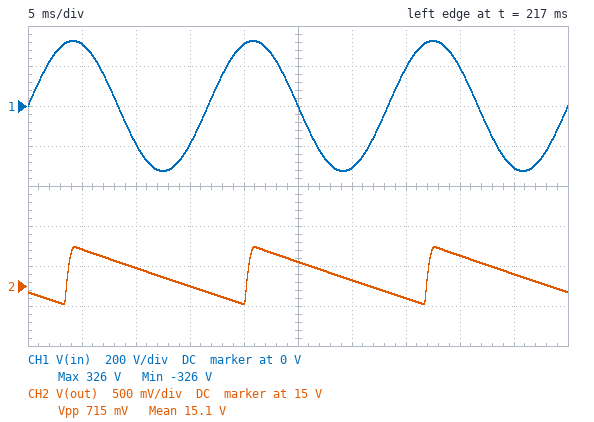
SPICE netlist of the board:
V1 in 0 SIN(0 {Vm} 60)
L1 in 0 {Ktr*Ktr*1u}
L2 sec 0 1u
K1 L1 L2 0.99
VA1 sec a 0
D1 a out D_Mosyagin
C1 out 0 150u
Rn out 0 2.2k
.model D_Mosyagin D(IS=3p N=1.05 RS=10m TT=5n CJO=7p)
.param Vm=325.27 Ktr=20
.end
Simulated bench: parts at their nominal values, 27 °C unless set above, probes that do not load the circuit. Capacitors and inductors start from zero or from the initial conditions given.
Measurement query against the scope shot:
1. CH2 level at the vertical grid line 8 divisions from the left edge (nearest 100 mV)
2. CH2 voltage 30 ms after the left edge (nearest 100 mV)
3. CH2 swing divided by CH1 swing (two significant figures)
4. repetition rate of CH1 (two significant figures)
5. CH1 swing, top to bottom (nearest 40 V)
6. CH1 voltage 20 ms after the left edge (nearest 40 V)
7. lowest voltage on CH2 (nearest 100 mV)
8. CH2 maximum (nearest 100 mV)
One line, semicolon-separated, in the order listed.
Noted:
15.4 V; 15.1 V; 0.0011; 60 Hz; 640 V; 320 V; 14.8 V; 15.5 V
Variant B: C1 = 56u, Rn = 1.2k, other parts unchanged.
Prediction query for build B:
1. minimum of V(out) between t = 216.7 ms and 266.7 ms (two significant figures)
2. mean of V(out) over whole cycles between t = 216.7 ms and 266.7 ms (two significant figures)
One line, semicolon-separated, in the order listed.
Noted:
12 V; 14 V
